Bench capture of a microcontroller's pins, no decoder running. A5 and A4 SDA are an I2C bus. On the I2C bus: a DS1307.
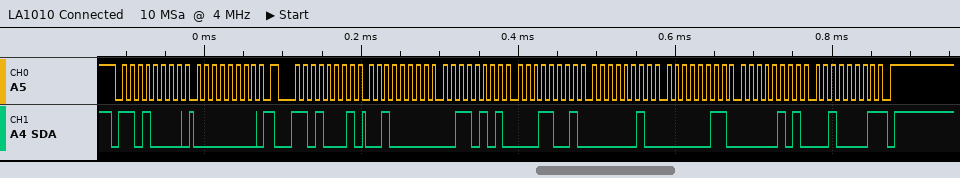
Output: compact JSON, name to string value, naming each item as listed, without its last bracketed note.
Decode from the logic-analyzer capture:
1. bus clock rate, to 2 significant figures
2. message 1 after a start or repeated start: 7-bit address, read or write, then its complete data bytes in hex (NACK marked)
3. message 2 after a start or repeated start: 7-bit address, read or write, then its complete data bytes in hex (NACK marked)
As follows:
{"bus clock rate, to 2 significant figures": "100 kHz", "message 1 after a start or repeated start: 7-bit address, read or write, then its complete data bytes in hex": "0x68 write: 00", "message 2 after a start or repeated start: 7-bit address, read or write, then its complete data bytes in hex": "0x68 read: 20 35 19 02 03 05 21 NACK"}
